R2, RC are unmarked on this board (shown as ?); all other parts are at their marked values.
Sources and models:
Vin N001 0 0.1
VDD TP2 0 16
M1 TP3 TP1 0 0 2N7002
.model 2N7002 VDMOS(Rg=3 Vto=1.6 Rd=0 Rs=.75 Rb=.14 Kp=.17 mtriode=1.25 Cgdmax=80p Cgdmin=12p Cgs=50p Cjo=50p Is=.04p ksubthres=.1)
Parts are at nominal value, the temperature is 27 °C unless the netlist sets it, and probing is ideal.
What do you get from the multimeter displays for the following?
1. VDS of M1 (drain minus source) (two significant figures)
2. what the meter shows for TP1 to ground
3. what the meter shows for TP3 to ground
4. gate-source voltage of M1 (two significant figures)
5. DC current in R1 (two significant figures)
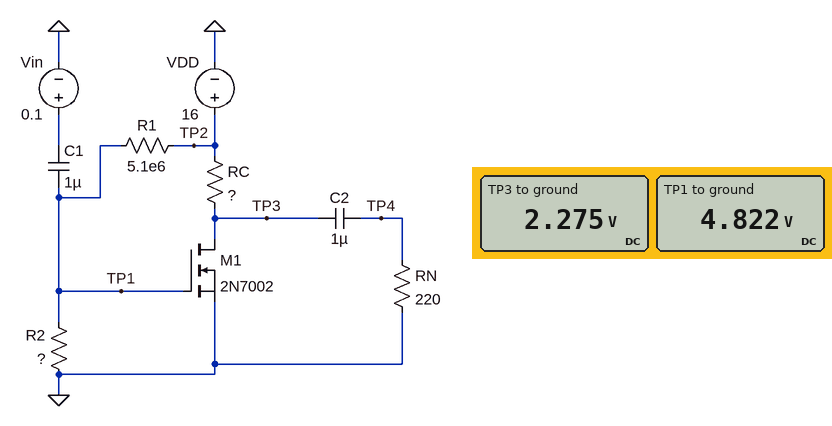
2.3 V
4.822 V
2.275 V
4.8 V
2.2 µA
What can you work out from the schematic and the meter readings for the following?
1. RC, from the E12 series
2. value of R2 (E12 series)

22 Ω
2.2 MΩ
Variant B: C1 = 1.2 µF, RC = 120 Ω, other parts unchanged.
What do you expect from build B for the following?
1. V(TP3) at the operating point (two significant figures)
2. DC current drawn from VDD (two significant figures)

300 mV
130 mA
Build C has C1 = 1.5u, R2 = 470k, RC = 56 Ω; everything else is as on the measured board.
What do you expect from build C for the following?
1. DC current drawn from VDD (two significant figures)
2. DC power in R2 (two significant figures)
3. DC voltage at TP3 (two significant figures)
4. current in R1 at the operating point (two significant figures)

8.2 µA
3.9 µW
16 V
2.9 µA
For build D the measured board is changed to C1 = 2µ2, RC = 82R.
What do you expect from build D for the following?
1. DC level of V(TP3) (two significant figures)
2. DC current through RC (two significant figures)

450 mV
190 mA
